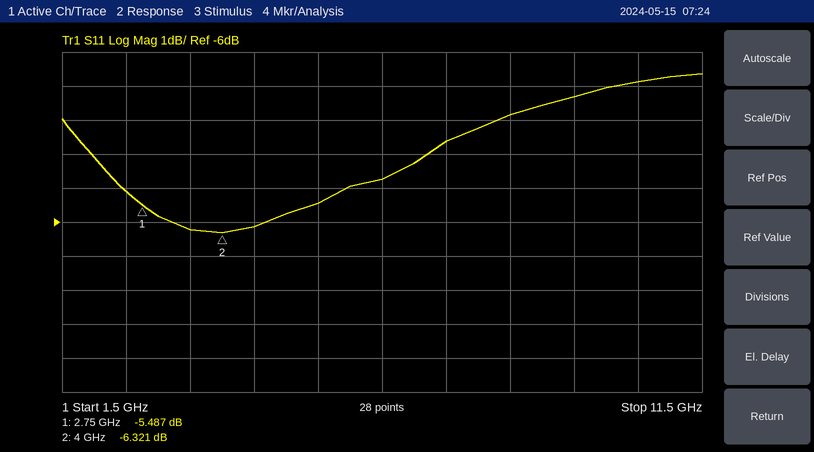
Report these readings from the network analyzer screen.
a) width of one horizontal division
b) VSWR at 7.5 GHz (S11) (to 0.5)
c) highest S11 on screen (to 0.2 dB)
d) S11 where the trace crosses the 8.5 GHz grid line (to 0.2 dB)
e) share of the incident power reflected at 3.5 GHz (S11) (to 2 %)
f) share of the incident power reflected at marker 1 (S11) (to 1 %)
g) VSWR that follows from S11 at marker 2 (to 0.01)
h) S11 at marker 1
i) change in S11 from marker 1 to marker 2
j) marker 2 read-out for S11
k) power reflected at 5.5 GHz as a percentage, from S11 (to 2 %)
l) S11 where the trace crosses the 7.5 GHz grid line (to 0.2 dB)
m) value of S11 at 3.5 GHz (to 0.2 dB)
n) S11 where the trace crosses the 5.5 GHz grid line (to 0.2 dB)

1 GHz
5.0
-1.6 dB
-2.8 dB
24 %
28 %
2.87
-5.487 dB
-0.834 dB
-6.321 dB
28 %
-3.6 dB
-6.2 dB
-5.4 dB
